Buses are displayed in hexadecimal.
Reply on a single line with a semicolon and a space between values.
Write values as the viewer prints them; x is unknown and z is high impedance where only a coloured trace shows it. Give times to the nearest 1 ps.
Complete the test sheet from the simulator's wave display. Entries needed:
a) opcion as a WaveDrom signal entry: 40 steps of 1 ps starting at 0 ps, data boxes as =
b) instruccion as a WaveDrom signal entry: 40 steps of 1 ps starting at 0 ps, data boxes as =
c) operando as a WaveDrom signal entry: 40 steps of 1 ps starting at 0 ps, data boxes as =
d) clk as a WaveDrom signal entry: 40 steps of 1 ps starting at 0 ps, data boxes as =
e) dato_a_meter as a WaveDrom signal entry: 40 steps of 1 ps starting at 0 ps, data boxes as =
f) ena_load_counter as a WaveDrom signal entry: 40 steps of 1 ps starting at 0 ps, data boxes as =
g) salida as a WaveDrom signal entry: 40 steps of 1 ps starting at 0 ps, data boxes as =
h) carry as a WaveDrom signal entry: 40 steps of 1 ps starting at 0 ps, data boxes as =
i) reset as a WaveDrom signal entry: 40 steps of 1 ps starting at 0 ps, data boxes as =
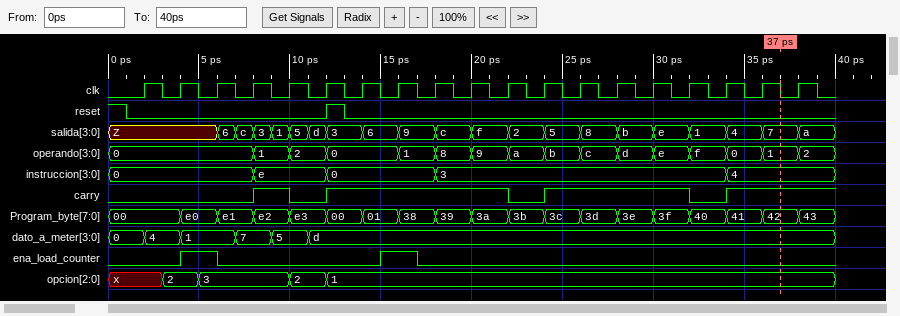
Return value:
{name: 'opcion', wave: 'x..=.=....=.=...........................', data: '2 3 2 1'}; {name: 'instruccion', wave: '=.......=...=.....=...............=.....', data: '0 e 0 3 4'}; {name: 'operando', wave: '=.......=.=.=...=.=.=.=.=.=.=.=.=.=.=.=.', data: '0 1 2 0 1 8 9 a b c d e f 0 1 2'}; {name: 'clk', wave: '0.10101010101010101010101010101010101010'}; {name: 'dato_a_meter', wave: '=.=.=..=.=.=............................', data: '0 4 1 7 5 d'}; {name: 'ena_load_counter', wave: '0...1.0........1.0......................'}; {name: 'salida', wave: '=.....=======.=.=.=.=.=.=.=.=.=.=.=.=.=.', data: 'Z 6 c 3 1 5 d 3 6 9 c f 2 5 8 b e 1 4 7 a'}; {name: 'carry', wave: '0.......1.0.1.........0.1.......0.1.....'}; {name: 'reset', wave: '10..........10..........................'}
